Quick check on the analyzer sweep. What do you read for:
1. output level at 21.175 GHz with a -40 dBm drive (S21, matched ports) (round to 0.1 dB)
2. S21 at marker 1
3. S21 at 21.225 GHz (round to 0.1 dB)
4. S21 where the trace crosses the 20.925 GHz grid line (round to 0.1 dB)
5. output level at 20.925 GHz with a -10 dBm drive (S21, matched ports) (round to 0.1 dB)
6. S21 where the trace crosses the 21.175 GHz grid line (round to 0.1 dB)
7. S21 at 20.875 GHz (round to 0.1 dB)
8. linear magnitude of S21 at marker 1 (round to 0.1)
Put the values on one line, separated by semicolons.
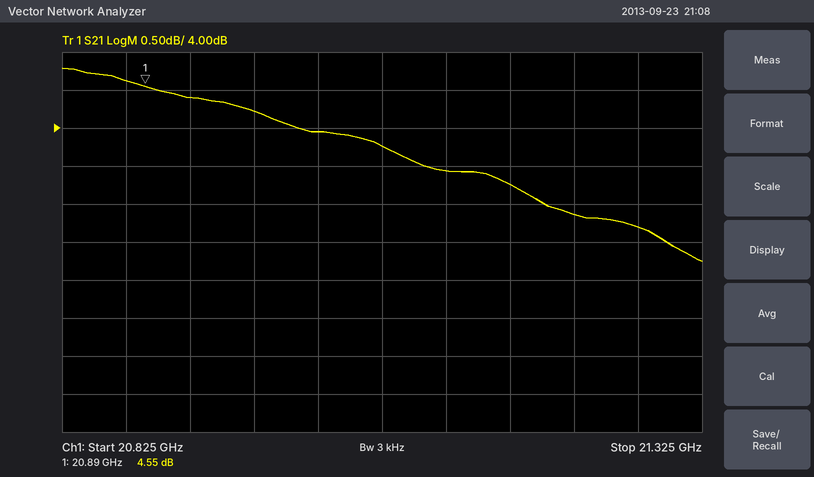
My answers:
-36.7 dBm; 4.55 dB; 2.9 dB; 4.4 dB; -5.6 dBm; 3.3 dB; 4.6 dB; 1.7
